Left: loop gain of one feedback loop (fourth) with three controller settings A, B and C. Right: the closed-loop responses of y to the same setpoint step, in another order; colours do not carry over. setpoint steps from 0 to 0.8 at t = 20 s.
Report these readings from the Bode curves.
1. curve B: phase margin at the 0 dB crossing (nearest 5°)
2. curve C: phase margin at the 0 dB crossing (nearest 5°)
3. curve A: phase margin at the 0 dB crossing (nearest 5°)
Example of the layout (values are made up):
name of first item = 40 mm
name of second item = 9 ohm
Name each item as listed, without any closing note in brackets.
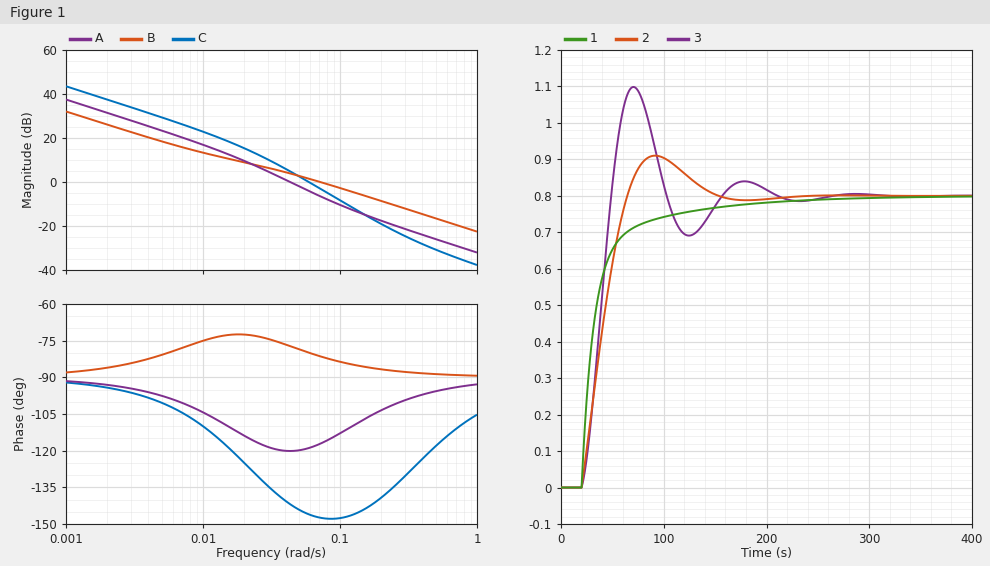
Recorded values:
curve B: phase margin at the 0 dB crossing = 100°
curve C: phase margin at the 0 dB crossing = 35°
curve A: phase margin at the 0 dB crossing = 60°
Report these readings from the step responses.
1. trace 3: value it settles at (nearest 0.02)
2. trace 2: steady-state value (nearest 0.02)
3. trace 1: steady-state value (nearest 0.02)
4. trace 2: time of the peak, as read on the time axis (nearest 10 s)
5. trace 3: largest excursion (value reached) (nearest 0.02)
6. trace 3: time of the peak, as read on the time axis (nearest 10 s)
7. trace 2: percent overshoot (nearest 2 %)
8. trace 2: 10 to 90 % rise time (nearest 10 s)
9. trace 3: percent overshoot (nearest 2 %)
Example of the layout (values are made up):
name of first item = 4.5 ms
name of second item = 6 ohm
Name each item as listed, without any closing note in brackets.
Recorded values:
trace 3: value it settles at = 0.80
trace 2: steady-state value = 0.80
trace 1: steady-state value = 0.80
trace 2: time of the peak, as read on the time axis = 90 s
trace 3: largest excursion (value reached) = 1.10
trace 3: time of the peak, as read on the time axis = 70 s
trace 2: percent overshoot = 14 %
trace 2: 10 to 90 % rise time = 30 s
trace 3: percent overshoot = 38 %
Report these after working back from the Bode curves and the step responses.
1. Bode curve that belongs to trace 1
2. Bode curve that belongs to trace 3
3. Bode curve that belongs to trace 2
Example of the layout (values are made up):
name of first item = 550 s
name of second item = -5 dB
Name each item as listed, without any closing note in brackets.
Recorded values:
Bode curve that belongs to trace 1 = B
Bode curve that belongs to trace 3 = C
Bode curve that belongs to trace 2 = A
